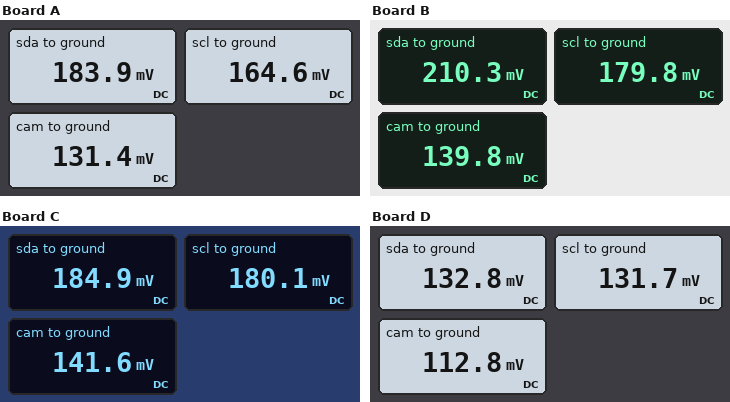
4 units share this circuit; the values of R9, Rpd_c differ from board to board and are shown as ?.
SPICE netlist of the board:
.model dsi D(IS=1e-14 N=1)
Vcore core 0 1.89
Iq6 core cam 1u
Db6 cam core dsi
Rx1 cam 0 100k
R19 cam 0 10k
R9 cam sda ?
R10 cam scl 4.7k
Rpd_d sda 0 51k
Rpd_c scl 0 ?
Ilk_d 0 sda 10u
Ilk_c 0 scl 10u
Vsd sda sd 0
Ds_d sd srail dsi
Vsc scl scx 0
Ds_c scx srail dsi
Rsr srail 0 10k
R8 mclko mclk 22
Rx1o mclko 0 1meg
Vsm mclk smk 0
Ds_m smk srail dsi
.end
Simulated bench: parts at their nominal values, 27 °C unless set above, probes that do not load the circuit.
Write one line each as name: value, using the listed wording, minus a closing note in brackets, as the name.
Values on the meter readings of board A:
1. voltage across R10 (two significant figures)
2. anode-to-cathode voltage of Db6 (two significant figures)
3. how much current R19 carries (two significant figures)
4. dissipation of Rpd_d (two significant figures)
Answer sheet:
voltage across R10: 33 mV
anode-to-cathode voltage of Db6: -1.8 V
how much current R19 carries: 13 µA
dissipation of Rpd_d: 660 nW
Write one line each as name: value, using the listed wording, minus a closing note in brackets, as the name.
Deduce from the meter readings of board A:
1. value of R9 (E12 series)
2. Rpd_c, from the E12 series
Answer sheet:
value of R9: 8.2 kΩ
Rpd_c, from the E12 series: 56 kΩ
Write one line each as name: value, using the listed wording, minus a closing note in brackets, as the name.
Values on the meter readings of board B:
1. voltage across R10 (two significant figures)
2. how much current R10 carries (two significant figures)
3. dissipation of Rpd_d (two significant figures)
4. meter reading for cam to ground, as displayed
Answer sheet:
voltage across R10: 40 mV
how much current R10 carries: 8.5 µA
dissipation of Rpd_d: 870 nW
meter reading for cam to ground, as displayed: 139.8 mV
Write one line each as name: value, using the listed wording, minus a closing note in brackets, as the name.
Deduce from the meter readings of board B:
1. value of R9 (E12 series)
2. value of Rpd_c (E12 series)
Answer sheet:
value of R9: 12 kΩ
value of Rpd_c: 120 kΩ
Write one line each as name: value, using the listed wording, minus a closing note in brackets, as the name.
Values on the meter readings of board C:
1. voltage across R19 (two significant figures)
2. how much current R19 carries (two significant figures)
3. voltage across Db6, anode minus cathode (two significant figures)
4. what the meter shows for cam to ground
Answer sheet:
voltage across R19: 140 mV
how much current R19 carries: 14 µA
voltage across Db6, anode minus cathode: -1.7 V
what the meter shows for cam to ground: 141.6 mV
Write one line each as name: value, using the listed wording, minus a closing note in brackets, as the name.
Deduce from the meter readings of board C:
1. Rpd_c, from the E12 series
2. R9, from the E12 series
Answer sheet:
Rpd_c, from the E12 series: 100 kΩ
R9, from the E12 series: 6.8 kΩ
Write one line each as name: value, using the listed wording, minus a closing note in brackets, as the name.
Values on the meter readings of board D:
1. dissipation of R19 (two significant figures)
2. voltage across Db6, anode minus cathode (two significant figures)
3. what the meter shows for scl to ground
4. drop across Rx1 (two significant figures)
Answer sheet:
dissipation of R19: 1.3 µW
voltage across Db6, anode minus cathode: -1.8 V
what the meter shows for scl to ground: 131.7 mV
drop across Rx1: 110 mV
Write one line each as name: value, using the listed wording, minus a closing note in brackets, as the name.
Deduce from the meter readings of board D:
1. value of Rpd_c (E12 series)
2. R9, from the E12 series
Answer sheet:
value of Rpd_c: 22 kΩ
R9, from the E12 series: 2.7 kΩ
